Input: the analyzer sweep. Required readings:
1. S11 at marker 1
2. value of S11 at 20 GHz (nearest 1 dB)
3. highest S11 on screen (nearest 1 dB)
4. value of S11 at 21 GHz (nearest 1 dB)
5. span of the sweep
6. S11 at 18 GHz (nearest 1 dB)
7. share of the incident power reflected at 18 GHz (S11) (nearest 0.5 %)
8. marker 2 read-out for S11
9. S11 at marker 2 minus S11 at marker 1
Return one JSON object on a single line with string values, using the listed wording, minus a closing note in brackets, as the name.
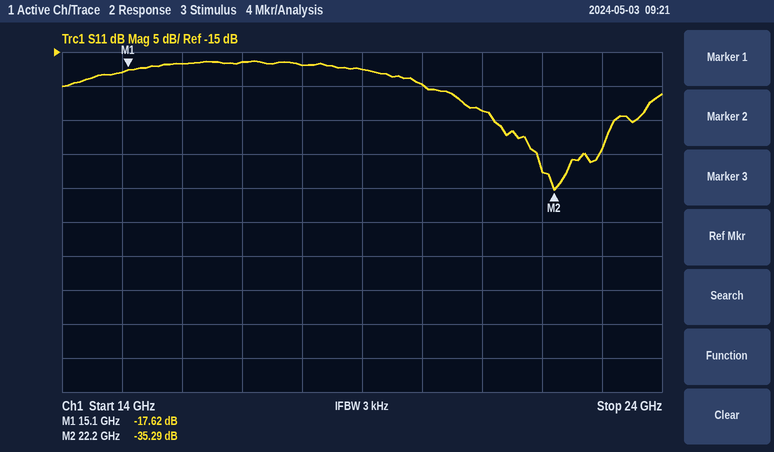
{"S11 at marker 1": "-17.62 dB", "value of S11 at 20 GHz": "-20 dB", "highest S11 on screen": "-16 dB", "value of S11 at 21 GHz": "-24 dB", "span of the sweep": "10 GHz", "S11 at 18 GHz": "-17 dB", "share of the incident power reflected at 18 GHz (S11)": "2.0 %", "marker 2 read-out for S11": "-35.29 dB", "S11 at marker 2 minus S11 at marker 1": "-17.67 dB"}
